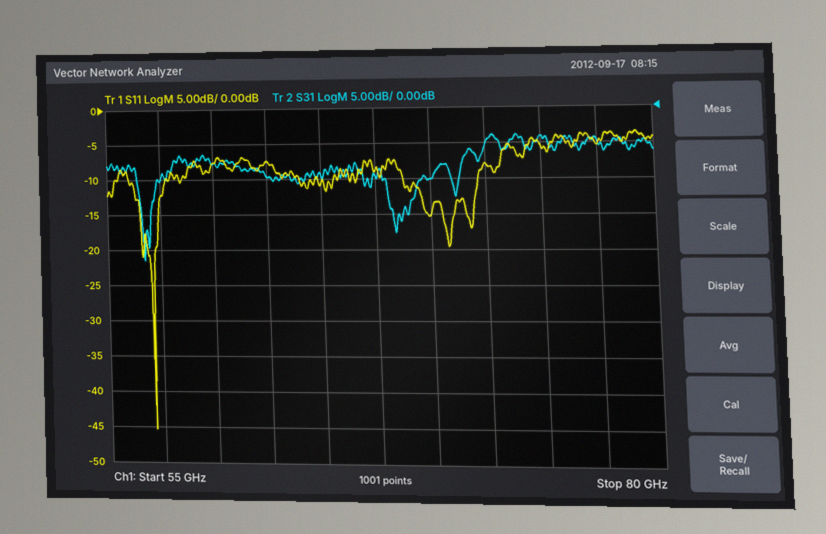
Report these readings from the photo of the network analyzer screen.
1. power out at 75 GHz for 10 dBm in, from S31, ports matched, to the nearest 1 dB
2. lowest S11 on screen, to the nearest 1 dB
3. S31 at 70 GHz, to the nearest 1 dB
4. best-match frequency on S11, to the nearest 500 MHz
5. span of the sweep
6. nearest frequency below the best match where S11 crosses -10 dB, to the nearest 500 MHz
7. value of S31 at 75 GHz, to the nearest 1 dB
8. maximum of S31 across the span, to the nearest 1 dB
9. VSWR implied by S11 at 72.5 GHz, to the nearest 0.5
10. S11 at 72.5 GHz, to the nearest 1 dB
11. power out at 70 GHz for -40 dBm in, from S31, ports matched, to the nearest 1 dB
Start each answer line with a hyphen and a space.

- 6 dBm
- -45 dB
- -10 dB
- 57.0 GHz
- 25 GHz
- 56.0 GHz
- -4 dB
- -4 dB
- 2.5
- -8 dB
- -50 dBm
